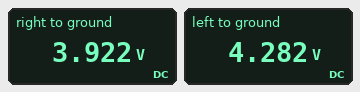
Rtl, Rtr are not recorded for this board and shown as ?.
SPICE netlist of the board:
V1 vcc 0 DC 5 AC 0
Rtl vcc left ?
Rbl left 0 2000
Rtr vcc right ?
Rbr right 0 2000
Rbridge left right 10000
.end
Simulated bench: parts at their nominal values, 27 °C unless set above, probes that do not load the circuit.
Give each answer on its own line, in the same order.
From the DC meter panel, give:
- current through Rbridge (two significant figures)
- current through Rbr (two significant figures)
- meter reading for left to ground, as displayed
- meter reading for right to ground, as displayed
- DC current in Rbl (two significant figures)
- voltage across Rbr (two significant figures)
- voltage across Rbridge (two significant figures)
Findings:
36 µA
2.0 mA
4.282 V
3.922 V
2.1 mA
3.9 V
360 mV
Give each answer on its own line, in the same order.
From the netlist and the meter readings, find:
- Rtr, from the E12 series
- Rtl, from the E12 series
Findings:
560 Ω
330 Ω
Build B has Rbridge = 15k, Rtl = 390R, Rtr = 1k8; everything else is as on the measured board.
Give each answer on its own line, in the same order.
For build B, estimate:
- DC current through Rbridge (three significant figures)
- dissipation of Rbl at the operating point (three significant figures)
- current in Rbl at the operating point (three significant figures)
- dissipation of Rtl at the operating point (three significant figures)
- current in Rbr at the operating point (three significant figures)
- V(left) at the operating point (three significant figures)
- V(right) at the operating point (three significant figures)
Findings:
95.4 µA
8.62 mW
2.08 mA
1.84 mW
1.36 mA
4.15 V
2.72 V
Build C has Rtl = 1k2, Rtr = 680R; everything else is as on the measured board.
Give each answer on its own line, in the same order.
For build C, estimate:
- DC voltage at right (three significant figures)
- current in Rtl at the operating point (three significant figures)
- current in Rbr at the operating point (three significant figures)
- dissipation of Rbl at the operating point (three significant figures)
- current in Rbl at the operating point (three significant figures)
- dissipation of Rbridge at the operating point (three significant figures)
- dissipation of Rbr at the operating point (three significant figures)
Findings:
3.70 V
1.53 mA
1.85 mA
5.01 mW
1.58 mA
29.0 µW
6.86 mW
